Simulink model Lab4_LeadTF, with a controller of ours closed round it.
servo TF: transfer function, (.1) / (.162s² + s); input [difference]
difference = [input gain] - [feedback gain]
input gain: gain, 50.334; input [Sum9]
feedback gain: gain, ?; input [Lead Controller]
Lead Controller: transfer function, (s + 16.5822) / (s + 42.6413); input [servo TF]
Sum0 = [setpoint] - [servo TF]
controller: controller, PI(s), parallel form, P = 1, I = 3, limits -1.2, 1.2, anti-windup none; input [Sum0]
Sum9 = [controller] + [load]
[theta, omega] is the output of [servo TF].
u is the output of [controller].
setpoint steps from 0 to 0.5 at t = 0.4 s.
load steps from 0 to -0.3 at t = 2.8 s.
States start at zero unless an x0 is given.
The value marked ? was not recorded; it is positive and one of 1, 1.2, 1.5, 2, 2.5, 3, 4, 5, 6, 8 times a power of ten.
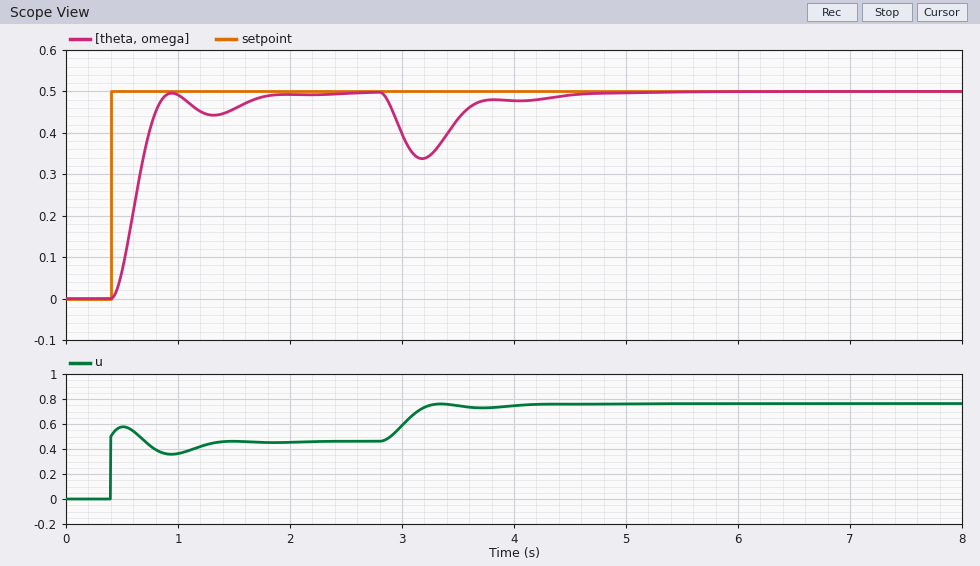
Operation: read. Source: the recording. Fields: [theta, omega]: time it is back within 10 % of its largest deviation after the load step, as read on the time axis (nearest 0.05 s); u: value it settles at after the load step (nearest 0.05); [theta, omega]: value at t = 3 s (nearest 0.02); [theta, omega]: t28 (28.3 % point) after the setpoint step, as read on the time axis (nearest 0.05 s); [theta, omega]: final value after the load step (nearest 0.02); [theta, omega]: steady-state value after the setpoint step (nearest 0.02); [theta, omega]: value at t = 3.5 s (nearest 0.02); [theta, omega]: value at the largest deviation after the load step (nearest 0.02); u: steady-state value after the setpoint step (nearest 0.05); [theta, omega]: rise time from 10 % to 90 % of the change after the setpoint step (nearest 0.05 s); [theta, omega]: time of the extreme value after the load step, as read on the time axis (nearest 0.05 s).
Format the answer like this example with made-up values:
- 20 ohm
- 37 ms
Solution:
- 4.30 s
- 0.75
- 0.40
- 0.55 s
- 0.50
- 0.50
- 0.44
- 0.34
- 0.45
- 0.30 s
- 3.20 s
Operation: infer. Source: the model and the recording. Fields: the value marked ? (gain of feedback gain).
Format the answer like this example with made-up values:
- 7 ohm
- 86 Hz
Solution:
- 120
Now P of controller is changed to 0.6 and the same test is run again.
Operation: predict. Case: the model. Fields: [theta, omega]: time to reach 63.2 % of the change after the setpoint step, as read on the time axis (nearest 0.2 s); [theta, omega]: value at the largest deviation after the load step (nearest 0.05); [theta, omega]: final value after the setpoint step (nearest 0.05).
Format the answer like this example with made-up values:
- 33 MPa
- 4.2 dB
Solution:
- 0.8 s
- 0.30
- 0.50
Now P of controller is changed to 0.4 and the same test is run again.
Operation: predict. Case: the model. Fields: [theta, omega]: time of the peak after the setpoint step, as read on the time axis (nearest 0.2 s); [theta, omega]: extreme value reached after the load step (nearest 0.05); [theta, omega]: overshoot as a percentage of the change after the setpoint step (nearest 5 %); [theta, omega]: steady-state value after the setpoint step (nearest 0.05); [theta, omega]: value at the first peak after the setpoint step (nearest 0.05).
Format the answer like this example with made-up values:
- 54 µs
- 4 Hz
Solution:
- 1.2 s
- 0.30
- 10 %
- 0.50
- 0.55
